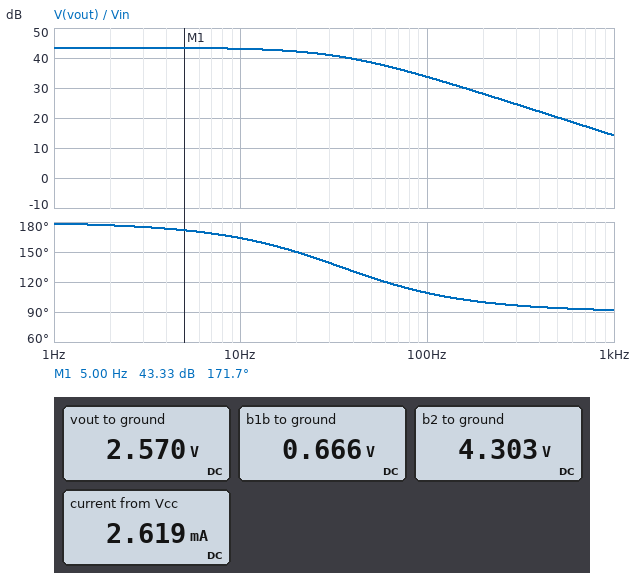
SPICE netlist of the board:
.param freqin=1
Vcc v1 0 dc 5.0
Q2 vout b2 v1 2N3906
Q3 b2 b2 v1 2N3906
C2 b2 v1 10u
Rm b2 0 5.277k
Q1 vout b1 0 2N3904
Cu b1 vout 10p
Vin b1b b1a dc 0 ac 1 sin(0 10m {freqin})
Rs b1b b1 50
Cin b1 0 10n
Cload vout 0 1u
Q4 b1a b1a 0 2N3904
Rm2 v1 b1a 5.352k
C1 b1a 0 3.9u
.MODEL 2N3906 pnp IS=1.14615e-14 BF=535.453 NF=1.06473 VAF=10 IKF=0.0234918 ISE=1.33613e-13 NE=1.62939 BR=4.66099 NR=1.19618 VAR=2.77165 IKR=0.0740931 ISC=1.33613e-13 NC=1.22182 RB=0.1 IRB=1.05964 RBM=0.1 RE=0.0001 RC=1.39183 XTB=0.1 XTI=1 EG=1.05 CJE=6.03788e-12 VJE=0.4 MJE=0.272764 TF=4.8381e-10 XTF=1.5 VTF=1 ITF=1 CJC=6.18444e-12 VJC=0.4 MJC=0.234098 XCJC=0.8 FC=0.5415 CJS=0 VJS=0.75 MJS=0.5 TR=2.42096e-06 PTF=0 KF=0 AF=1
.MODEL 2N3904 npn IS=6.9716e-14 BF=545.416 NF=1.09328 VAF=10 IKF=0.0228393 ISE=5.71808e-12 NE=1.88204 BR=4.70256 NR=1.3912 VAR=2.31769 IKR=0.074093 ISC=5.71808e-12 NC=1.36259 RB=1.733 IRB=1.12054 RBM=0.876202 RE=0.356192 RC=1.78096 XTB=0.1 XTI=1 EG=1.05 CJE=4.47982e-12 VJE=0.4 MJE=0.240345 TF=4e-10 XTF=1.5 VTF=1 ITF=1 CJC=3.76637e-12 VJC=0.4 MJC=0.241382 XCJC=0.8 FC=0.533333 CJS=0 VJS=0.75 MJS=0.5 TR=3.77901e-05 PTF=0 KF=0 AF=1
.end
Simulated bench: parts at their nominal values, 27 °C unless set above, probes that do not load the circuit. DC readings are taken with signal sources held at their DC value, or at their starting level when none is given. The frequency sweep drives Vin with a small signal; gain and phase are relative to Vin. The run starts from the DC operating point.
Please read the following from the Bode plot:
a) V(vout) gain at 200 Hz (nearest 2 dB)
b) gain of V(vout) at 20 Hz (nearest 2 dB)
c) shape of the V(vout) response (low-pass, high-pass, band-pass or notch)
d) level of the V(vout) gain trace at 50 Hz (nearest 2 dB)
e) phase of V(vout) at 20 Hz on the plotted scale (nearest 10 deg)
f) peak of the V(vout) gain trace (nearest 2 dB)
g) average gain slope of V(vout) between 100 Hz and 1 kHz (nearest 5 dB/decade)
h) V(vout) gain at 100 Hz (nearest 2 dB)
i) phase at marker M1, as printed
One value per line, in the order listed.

28 dB
42 dB
low-pass
38 dB
150 deg
44 dB
-20 dB/decade
34 dB
171.7 deg
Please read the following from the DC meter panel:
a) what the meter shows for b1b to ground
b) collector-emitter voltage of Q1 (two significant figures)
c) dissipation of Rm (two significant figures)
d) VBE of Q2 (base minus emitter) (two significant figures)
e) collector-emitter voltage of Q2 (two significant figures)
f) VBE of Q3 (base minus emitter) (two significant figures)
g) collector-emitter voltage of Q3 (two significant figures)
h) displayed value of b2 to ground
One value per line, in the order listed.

0.666 V
2.6 V
3.5 mW
-700 mV
-2.4 V
-700 mV
-700 mV
4.303 V
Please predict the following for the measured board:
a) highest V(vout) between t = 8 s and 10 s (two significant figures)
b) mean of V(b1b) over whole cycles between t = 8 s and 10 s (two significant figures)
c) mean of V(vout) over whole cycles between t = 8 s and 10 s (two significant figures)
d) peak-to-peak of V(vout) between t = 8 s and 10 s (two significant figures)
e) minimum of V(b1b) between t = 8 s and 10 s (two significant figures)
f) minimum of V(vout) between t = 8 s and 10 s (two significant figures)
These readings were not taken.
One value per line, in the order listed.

4.1 V
670 mV
2.6 V
2.9 V
660 mV
1.1 V
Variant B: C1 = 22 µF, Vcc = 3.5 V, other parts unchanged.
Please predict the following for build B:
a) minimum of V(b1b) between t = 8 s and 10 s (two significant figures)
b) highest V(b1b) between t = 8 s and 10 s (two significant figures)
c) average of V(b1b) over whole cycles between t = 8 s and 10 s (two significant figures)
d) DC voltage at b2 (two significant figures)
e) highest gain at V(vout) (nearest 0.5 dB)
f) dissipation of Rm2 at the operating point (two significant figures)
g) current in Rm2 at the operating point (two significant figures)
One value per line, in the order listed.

640 mV
660 mV
650 mV
2.8 V
43.0 dB
1.5 mW
530 µA
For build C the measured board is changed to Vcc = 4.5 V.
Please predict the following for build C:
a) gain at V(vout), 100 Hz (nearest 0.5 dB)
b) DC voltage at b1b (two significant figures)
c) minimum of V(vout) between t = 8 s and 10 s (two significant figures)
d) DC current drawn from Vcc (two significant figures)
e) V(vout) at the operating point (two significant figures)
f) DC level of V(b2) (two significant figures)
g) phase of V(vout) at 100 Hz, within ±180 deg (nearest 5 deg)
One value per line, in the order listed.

32.5 dB
660 mV
890 mV
2.3 mA
2.3 V
3.8 V
105 deg
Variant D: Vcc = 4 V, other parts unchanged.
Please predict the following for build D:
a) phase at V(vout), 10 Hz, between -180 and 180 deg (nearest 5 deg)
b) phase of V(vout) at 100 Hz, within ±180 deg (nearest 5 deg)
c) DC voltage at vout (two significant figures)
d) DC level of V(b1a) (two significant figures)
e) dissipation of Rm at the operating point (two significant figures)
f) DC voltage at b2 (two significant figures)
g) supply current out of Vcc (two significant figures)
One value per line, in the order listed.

160 deg
105 deg
2.1 V
660 mV
2.1 mW
3.3 V
2.0 mA
